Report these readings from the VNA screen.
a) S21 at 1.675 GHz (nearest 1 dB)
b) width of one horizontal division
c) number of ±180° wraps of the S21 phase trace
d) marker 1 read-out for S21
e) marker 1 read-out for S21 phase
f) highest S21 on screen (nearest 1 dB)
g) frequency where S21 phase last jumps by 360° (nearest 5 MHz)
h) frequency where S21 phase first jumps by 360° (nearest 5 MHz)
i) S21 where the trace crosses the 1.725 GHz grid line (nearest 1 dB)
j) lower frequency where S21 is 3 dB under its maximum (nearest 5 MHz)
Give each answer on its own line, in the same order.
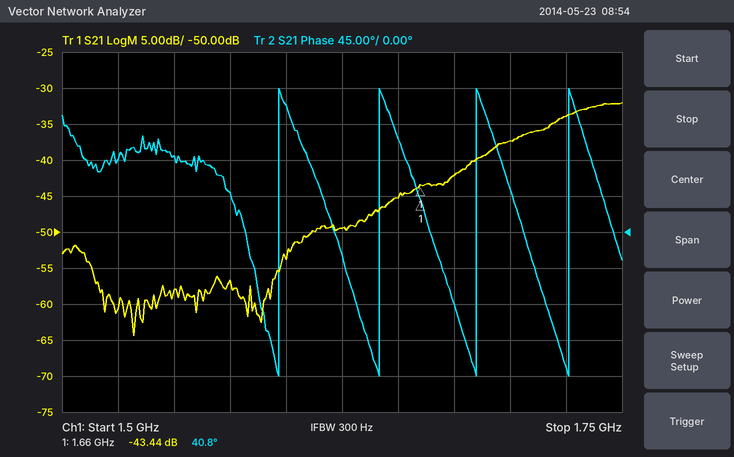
-42 dB
25 MHz
4
-43.44 dB
40.8°
-32 dB
1.725 GHz
1.595 GHz
-34 dB
1.720 GHz
